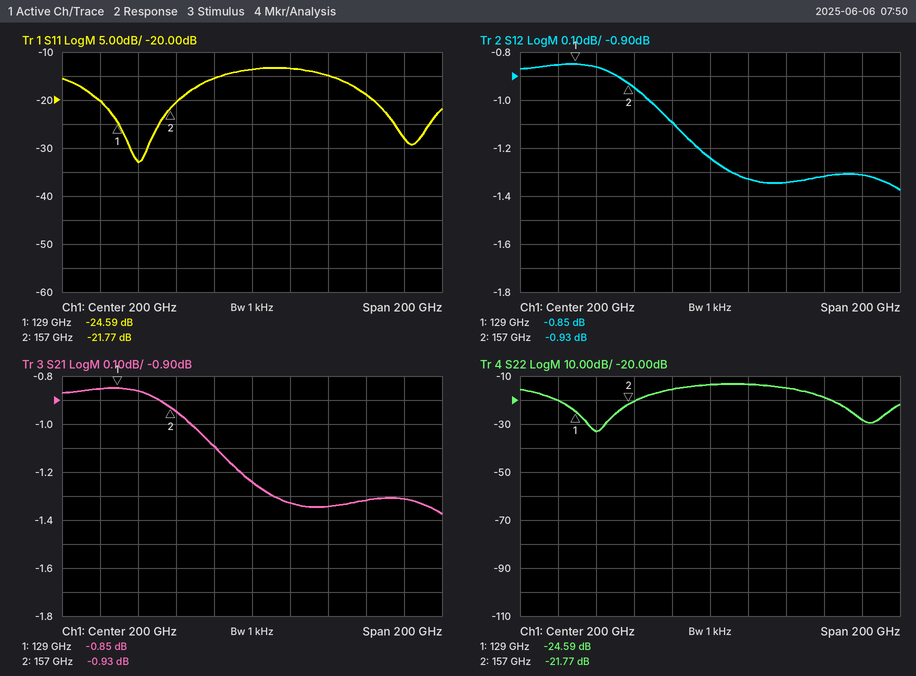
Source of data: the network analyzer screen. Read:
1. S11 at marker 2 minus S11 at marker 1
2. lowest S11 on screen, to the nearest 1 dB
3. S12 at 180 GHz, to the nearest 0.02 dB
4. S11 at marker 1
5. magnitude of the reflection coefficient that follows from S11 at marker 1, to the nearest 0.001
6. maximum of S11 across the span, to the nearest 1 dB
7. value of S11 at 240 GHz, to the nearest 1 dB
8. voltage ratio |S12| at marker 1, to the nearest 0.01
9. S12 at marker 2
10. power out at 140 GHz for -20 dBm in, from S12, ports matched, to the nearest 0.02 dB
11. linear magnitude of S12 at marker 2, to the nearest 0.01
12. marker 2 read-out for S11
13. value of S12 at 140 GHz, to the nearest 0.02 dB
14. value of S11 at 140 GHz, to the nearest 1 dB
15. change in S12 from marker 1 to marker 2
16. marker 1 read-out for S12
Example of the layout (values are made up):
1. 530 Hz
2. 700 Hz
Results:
1. 2.82 dB
2. -33 dB
3. -1.10 dB
4. -24.59 dB
5. 0.059
6. -13 dB
7. -15 dB
8. 0.91
9. -0.93 dB
10. -20.86 dBm
11. 0.90
12. -21.77 dB
13. -0.86 dB
14. -33 dB
15. -0.08 dB
16. -0.85 dB
